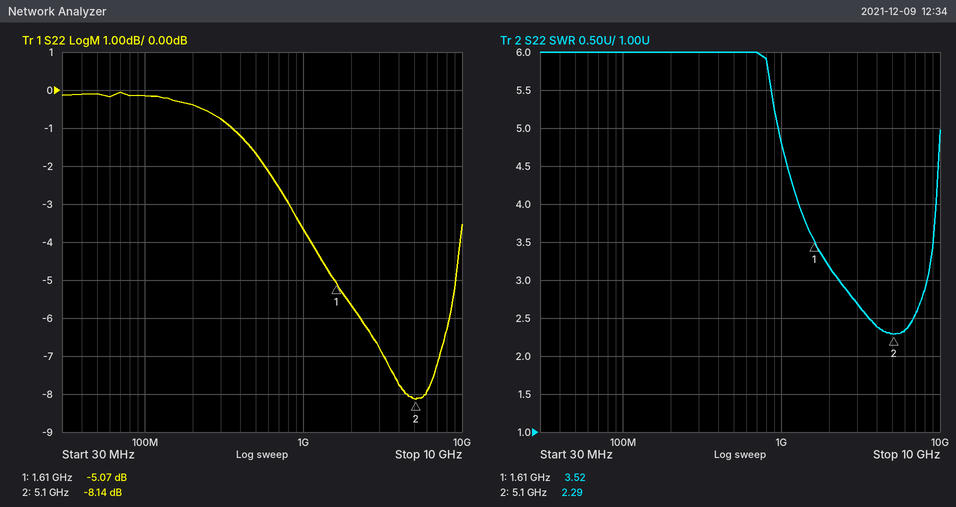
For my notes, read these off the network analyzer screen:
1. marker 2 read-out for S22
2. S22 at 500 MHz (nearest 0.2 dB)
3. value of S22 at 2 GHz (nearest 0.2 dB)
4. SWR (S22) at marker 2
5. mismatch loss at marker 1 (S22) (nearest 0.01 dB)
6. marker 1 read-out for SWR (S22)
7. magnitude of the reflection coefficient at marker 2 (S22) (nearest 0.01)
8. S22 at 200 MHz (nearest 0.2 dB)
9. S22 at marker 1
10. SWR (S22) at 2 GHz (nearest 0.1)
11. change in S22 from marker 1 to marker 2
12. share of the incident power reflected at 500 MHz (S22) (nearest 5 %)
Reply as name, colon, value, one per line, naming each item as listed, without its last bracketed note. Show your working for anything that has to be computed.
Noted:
marker 2 read-out for S22: -8.14 dB
S22 at 500 MHz: -1.6 dB
value of S22 at 2 GHz: -5.6 dB
SWR (S22) at marker 2: 2.29
mismatch loss at marker 1 (S22): −10 log10(1 − 10^(-5.07/10)) ≈ 1.62 dB
marker 1 read-out for SWR: 3.52
magnitude of the reflection coefficient at marker 2 (S22): 10^(-8.14/20) ≈ 0.39
S22 at 200 MHz: -0.4 dB
S22 at marker 1: -5.07 dB
SWR (S22) at 2 GHz: 3.2
change in S22 from marker 1 to marker 2: -8.14 − (-5.07) = -3.07 dB
share of the incident power reflected at 500 MHz (S22): 10^(-1.6/10) ≈ 69.2 %, so 70 % to the nearest 5 %
